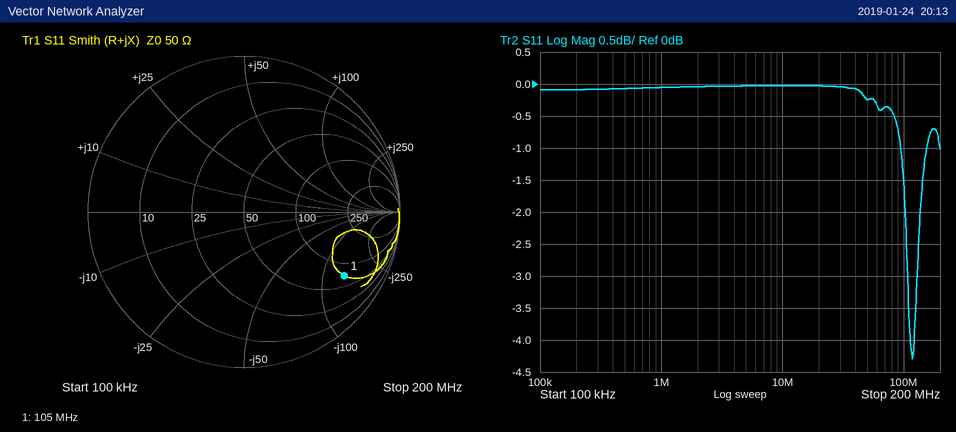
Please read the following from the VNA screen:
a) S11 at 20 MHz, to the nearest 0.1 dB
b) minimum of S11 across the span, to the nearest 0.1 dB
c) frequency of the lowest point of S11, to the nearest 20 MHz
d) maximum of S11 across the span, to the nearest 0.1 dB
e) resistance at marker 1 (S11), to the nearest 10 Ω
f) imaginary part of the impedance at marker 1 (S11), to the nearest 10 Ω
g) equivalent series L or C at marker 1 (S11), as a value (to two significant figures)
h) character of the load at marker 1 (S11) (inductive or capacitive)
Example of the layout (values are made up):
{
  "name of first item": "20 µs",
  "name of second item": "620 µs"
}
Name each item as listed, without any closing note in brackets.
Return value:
{
  "S11 at 20 MHz, to the nearest 0.1 dB": "0.0 dB",
  "minimum of S11 across the span, to the nearest 0.1 dB": "-4.3 dB",
  "frequency of the lowest point of S11, to the nearest 20 MHz": "120 MHz",
  "maximum of S11 across the span, to the nearest 0.1 dB": "0.0 dB",
  "resistance at marker 1 (S11), to the nearest 10 Ω": "70 Ω",
  "imaginary part of the impedance at marker 1 (S11), to the nearest 10 Ω": "-140 Ω",
  "equivalent series L or C at marker 1 (S11), as a value": "11 pF",
  "character of the load at marker 1 (S11)": "capacitive"
}
